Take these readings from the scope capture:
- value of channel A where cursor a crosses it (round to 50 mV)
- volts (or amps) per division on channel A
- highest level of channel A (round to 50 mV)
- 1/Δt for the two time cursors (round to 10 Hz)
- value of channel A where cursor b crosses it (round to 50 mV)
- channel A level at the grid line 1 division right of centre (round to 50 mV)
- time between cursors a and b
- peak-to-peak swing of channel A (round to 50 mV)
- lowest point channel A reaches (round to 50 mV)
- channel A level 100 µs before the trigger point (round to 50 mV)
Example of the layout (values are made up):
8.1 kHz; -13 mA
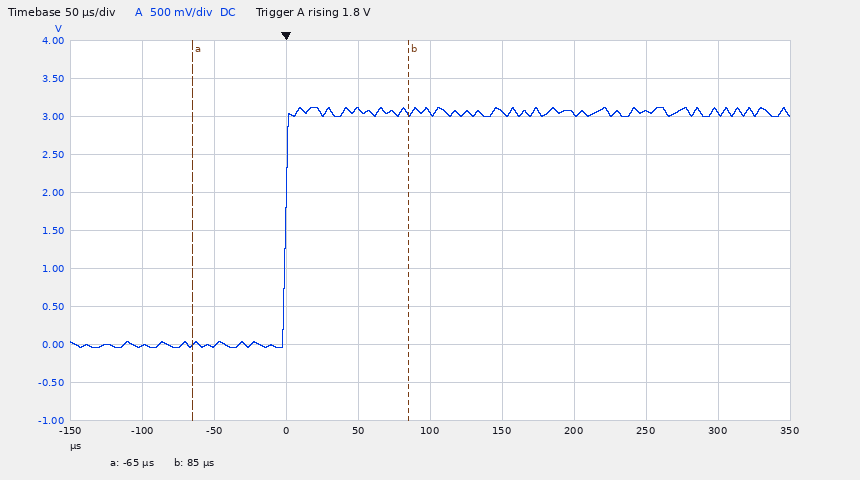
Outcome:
0 mV; 500 mV; 3.10 V; 6.67 kHz; 3.05 V; 3.05 V; 150 µs; 3.15 V; -50 mV; 0 mV
